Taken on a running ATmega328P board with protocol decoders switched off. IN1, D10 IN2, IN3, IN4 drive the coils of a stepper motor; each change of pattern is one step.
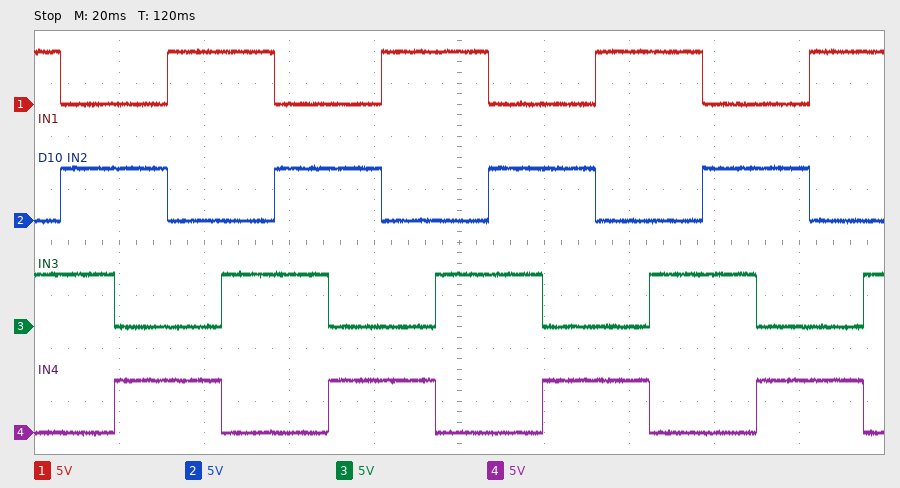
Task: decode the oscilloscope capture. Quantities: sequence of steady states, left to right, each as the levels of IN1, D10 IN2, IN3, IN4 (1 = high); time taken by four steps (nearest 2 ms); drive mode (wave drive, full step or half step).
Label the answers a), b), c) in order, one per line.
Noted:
a) 1010 0110 0101 1001 1010 0110 0101 1001 1010 0110 0101 1001 1010 0110 0101 1001 1010
b) 50 ms
c) full step
